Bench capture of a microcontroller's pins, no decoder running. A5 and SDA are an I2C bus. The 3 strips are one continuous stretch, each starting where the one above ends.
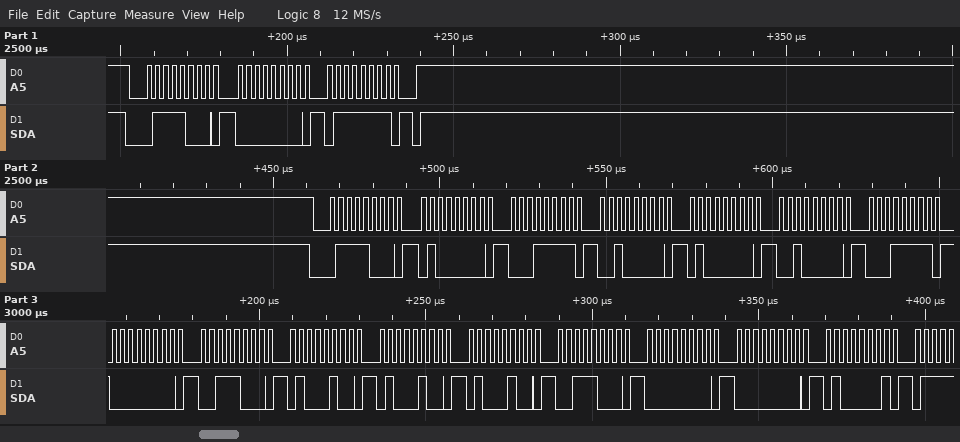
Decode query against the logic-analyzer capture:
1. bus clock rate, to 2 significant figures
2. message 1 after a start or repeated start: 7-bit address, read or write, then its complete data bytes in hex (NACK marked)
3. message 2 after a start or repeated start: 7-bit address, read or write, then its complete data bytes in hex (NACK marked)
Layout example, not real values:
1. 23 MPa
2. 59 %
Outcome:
1. 400 kHz
2. 0x3C write: 00 7F
3. 0x3C write: 40 1F 20 40 20 1F 00 38 44 44 44 38 00 00 41
